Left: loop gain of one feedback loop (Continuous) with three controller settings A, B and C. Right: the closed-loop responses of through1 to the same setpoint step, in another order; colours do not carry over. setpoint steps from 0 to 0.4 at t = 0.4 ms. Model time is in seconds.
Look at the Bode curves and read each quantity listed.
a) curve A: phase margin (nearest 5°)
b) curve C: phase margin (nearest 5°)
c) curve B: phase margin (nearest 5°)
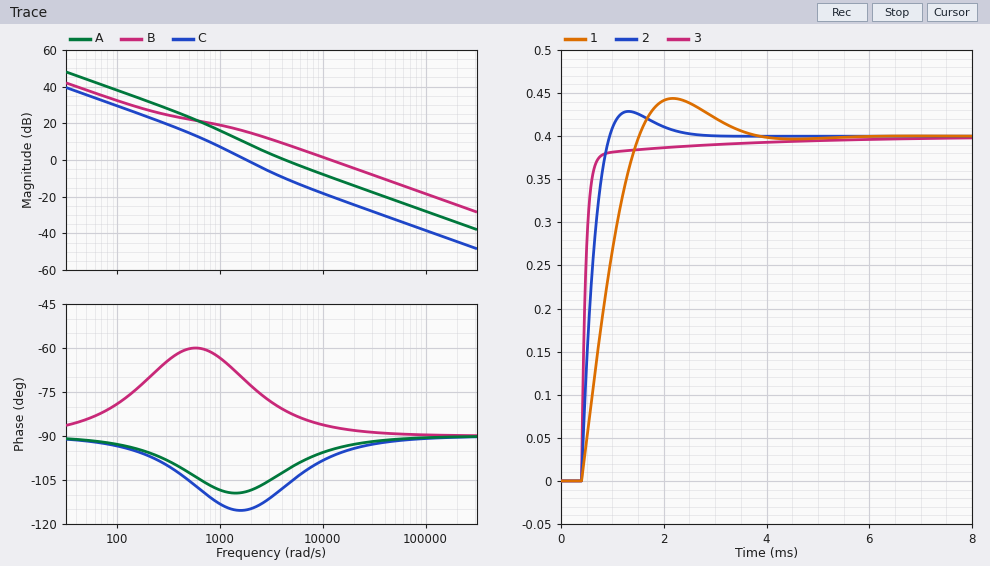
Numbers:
80°
65°
95°
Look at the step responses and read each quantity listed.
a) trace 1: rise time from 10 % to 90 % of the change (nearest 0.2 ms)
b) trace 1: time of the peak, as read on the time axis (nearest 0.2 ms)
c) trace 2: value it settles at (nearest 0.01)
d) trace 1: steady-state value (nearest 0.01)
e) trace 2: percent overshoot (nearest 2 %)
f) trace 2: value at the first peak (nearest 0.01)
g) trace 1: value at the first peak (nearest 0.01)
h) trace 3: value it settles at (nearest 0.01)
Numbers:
0.8 ms
2.2 ms
0.40
0.40
8 %
0.43
0.44
0.40
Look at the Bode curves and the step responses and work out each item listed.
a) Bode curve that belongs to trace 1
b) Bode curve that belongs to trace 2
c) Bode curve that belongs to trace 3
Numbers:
C
A
B
